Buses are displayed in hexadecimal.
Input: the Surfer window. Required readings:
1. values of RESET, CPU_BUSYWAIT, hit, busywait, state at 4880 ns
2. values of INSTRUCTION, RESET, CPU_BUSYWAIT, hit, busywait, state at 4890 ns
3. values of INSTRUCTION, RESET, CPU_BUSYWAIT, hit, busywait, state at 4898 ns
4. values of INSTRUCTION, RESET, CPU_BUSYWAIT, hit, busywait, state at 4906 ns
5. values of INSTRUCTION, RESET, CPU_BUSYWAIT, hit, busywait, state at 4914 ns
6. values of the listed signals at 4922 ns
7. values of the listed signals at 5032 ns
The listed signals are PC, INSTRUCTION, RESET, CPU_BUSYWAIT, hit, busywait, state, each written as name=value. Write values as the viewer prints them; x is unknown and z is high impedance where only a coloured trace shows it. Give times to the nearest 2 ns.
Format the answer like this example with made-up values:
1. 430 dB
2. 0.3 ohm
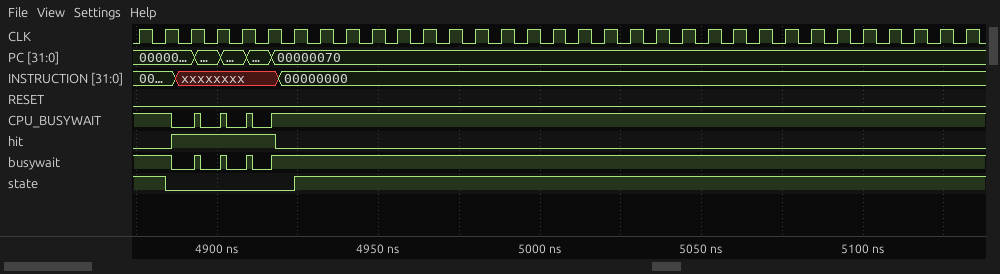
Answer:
1. RESET=0, CPU_BUSYWAIT=1, hit=0, busywait=1, state=1
2. INSTRUCTION=xxxxxxxx, RESET=0, CPU_BUSYWAIT=0, hit=1, busywait=0, state=0
3. INSTRUCTION=xxxxxxxx, RESET=0, CPU_BUSYWAIT=0, hit=1, busywait=0, state=0
4. INSTRUCTION=xxxxxxxx, RESET=0, CPU_BUSYWAIT=0, hit=1, busywait=0, state=0
5. INSTRUCTION=xxxxxxxx, RESET=0, CPU_BUSYWAIT=0, hit=1, busywait=0, state=0
6. PC=00000070, INSTRUCTION=00000000, RESET=0, CPU_BUSYWAIT=1, hit=0, busywait=1, state=0
7. PC=00000070, INSTRUCTION=00000000, RESET=0, CPU_BUSYWAIT=1, hit=0, busywait=1, state=1
